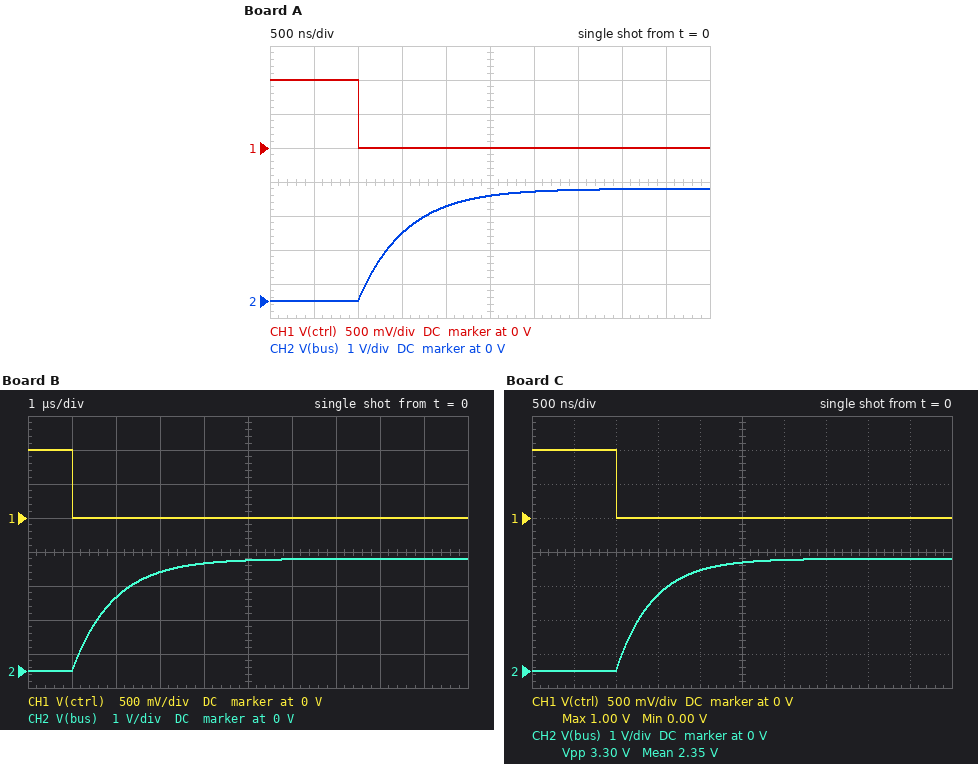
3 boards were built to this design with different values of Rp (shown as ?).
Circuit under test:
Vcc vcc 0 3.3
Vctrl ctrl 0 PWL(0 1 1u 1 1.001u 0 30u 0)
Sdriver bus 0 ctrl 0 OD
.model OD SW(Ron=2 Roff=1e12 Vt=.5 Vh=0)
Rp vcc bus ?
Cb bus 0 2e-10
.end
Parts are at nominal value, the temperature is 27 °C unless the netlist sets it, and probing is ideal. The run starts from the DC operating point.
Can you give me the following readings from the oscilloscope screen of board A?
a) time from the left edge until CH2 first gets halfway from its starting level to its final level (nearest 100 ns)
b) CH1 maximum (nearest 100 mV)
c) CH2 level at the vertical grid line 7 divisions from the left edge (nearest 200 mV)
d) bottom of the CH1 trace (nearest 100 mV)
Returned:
1.4 µs
1.0 V
3.2 V
0 V
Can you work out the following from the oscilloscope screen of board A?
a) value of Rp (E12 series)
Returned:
2.7 kΩ
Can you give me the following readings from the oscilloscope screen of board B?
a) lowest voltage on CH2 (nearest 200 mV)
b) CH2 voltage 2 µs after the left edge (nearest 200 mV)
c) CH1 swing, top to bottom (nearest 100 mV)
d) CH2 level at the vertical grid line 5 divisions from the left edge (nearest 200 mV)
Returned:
0 V
2.2 V
1.0 V
3.2 V
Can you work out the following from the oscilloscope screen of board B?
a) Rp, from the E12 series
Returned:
4.7 kΩ
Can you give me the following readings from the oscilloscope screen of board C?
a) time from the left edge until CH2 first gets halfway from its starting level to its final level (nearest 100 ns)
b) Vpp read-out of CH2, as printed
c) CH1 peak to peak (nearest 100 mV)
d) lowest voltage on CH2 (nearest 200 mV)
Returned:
1.3 µs
3.30 V
1.0 V
0 V
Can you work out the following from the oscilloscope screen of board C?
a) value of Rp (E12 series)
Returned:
2.2 kΩ
